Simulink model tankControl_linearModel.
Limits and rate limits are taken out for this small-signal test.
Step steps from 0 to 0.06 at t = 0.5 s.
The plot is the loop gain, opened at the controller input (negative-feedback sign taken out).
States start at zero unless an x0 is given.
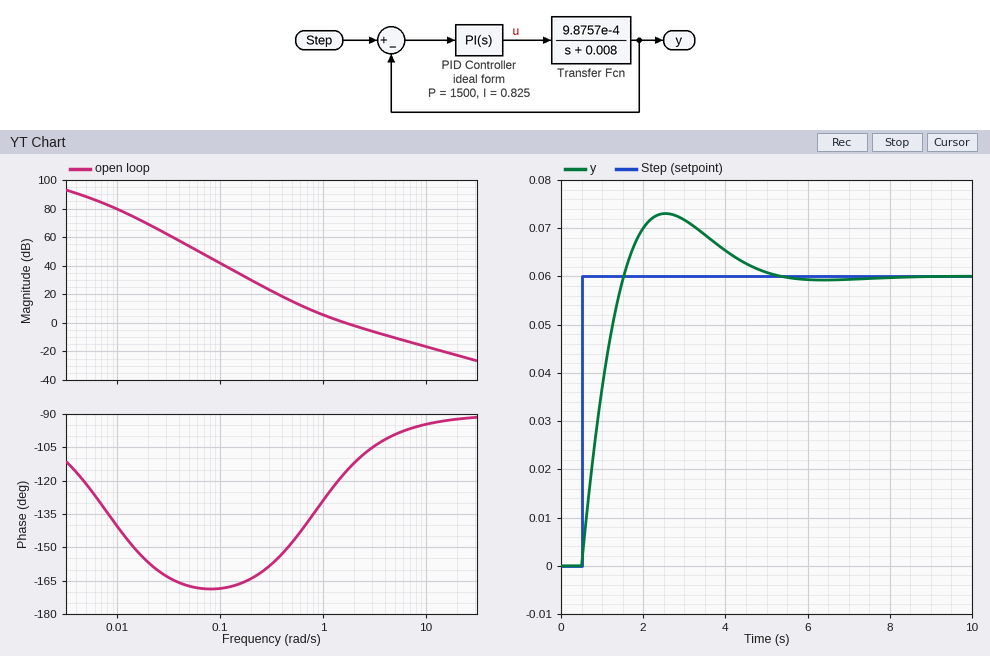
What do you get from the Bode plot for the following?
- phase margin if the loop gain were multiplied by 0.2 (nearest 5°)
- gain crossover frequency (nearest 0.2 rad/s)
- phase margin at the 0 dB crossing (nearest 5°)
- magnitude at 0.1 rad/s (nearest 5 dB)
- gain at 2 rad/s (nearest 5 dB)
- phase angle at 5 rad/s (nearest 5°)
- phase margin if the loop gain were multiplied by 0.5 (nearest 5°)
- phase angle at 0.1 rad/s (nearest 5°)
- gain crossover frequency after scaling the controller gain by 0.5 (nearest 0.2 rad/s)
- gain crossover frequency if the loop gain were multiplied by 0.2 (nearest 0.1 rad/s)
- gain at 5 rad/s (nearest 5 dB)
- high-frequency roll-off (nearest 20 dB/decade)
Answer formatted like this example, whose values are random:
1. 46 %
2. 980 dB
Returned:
1. 35°
2. 1.6 rad/s
3. 65°
4. 40 dB
5. 0 dB
6. -100°
7. 50°
8. -170°
9. 1.0 rad/s
10. 0.5 rad/s
11. -10 dB
12. -20 dB/decade
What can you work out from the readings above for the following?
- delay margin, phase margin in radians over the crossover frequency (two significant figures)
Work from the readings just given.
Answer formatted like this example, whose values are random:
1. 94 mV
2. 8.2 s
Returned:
1. 0.71 s
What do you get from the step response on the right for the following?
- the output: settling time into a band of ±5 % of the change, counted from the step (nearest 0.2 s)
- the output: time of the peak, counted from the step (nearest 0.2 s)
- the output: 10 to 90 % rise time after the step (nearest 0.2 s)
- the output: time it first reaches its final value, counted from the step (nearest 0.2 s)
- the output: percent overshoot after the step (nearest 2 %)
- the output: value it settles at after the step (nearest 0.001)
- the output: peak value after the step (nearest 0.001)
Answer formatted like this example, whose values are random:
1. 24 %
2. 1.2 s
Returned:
1. 4.0 s
2. 2.0 s
3. 0.8 s
4. 1.0 s
5. 22 %
6. 0.060
7. 0.073
